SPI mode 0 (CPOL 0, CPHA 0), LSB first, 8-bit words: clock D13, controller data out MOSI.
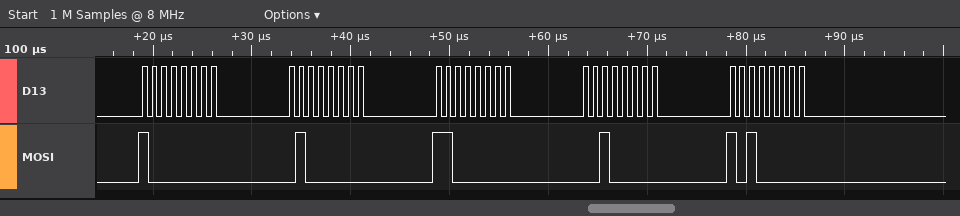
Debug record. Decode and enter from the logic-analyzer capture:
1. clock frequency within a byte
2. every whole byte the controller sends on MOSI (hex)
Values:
1 MHz
01 02 03 04 05
